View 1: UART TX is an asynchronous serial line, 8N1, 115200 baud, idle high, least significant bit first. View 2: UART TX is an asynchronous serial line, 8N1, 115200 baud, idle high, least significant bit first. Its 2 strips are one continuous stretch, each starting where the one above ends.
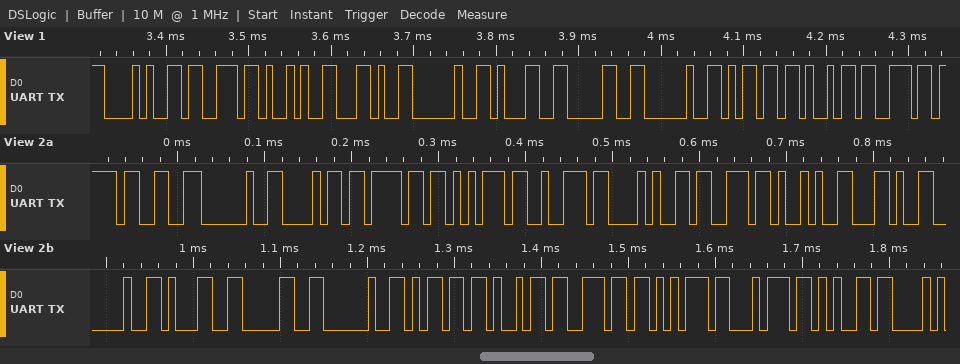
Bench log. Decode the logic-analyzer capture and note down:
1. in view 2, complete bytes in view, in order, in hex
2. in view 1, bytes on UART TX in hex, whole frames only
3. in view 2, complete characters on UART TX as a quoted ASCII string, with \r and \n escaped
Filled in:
0x33 0x20 0x68 0x6F 0x75 0x72 0x28 0x73 0x29 0x2C 0x20 0x31 0x30 0x20 0x6D 0x69 0x6E 0x75 0x74 0x65
28 73 29 2C 20 31 30 20 6D 69 6E
"3 hour(s), 10 minute"
